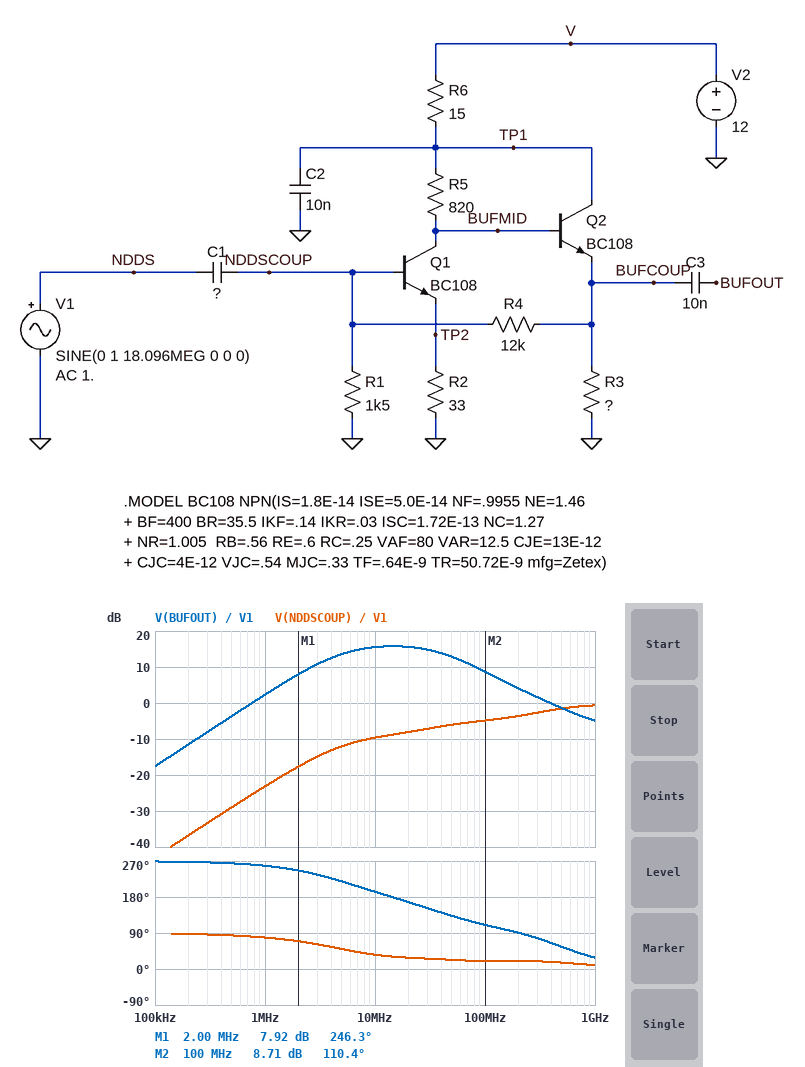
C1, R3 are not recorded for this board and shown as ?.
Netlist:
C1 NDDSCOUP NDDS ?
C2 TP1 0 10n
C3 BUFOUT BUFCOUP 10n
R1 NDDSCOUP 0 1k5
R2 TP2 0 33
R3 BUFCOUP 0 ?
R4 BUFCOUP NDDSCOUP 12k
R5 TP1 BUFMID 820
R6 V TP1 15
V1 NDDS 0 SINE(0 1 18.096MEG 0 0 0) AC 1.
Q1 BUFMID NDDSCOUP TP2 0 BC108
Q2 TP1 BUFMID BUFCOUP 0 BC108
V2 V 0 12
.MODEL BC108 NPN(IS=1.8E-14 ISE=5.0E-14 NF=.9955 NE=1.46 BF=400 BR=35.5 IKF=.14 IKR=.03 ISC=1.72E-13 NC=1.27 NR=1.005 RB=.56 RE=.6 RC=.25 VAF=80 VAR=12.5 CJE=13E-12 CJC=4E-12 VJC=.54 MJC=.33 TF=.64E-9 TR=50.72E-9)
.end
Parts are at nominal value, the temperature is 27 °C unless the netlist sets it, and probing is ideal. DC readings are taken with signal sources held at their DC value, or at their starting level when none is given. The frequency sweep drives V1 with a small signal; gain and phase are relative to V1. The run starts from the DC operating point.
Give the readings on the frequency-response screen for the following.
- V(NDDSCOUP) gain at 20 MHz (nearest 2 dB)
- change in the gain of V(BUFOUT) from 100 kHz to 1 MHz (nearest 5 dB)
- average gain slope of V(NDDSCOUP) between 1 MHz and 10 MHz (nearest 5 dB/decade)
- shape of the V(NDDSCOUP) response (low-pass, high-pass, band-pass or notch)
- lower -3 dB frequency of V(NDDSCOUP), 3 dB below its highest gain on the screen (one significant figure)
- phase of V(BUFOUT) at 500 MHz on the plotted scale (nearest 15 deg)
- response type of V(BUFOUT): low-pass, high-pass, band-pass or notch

-8 dB
20 dB
15 dB/decade
high-pass
200 MHz
60 deg
band-pass
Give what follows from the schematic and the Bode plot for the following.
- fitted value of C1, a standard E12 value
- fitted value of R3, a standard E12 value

27 pF
180 Ω
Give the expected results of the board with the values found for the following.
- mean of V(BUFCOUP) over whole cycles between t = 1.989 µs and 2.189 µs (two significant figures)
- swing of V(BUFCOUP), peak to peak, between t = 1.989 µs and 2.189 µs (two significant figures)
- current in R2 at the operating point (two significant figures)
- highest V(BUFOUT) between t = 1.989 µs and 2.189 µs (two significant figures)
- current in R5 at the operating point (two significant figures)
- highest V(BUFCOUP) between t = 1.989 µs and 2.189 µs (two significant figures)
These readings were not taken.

6.7 V
8.4 V
3.8 mA
2.9 V
3.9 mA
10 V
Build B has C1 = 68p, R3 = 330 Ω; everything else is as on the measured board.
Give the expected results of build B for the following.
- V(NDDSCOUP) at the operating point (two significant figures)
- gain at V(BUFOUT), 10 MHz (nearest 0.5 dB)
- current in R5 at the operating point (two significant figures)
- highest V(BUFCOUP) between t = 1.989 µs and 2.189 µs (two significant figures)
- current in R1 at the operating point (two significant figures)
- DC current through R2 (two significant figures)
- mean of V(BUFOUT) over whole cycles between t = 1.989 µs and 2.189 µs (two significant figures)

810 mV
20.5 dB
4.2 mA
11 V
540 µA
4.1 mA
-1.2 V
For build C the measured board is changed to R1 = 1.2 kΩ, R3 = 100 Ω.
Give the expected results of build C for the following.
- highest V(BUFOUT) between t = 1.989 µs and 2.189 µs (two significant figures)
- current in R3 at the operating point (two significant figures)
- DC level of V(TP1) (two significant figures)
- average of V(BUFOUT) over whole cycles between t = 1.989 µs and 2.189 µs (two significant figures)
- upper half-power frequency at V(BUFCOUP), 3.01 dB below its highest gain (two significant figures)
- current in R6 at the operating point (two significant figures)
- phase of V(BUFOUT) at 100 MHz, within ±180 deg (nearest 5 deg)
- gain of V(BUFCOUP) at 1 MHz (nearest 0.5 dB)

1.5 V
80 mA
11 V
-1.1 V
37 MHz
83 mA
105 deg
1.0 dB
